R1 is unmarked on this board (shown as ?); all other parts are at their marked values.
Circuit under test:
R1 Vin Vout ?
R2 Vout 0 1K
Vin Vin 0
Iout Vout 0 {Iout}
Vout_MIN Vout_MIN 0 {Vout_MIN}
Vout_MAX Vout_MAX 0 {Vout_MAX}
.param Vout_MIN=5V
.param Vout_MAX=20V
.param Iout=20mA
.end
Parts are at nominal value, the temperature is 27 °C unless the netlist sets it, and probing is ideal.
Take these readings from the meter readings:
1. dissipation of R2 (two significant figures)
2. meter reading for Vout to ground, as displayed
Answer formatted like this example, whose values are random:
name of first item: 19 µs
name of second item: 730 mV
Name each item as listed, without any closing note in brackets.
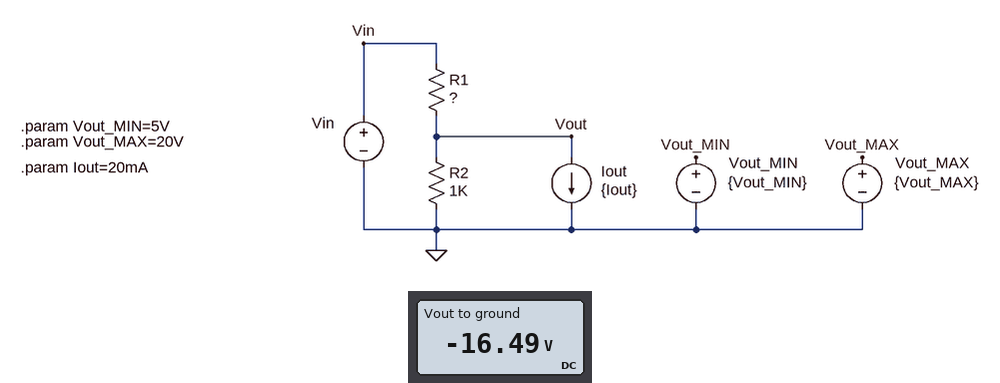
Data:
dissipation of R2: 270 mW
meter reading for Vout to ground, as displayed: -16.49 V
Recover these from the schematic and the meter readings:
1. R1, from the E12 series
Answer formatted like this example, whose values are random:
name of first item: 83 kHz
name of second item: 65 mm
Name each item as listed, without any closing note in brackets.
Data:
R1, from the E12 series: 4.7 kΩ
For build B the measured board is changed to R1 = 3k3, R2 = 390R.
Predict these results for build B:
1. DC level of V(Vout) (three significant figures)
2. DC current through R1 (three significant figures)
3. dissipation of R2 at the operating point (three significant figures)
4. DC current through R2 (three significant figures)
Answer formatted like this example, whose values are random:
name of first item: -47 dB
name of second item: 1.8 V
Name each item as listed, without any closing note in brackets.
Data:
DC level of V(Vout): -6.98 V
DC current through R1: 2.11 mA
dissipation of R2 at the operating point: 125 mW
DC current through R2: 17.9 mA
